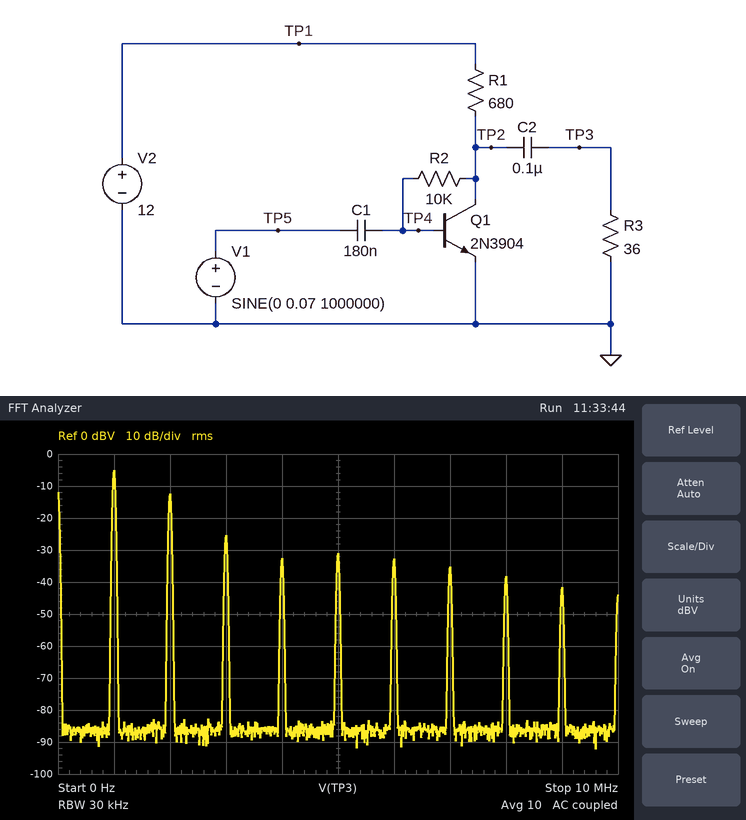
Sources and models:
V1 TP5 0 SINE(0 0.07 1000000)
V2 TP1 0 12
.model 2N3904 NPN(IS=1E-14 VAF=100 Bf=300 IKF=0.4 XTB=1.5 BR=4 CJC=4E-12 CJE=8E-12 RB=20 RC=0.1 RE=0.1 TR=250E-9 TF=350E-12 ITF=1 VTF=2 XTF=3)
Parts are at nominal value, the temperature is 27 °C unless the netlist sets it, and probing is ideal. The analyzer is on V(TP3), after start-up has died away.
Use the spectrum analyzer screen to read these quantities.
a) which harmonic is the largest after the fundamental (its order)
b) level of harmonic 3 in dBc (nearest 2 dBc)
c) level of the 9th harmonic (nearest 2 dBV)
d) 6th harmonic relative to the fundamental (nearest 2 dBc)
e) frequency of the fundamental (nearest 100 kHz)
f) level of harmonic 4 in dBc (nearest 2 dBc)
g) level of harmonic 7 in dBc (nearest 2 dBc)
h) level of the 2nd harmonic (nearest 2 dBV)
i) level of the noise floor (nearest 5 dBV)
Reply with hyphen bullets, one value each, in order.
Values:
- 2
- -20 dBc
- -42 dBV
- -28 dBc
- 1.0 MHz
- -28 dBc
- -30 dBc
- -12 dBV
- -85 dBV
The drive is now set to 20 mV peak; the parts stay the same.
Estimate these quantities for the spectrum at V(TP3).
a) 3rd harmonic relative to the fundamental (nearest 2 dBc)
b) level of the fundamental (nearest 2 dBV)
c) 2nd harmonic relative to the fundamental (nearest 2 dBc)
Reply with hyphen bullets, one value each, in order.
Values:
- -40 dBc
- -12 dBV
- -16 dBc
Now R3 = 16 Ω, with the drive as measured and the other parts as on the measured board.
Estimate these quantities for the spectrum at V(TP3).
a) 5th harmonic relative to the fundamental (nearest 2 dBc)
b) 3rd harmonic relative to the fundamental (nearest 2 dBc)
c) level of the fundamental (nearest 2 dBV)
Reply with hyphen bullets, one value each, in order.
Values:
- -44 dBc
- -18 dBc
- -12 dBV
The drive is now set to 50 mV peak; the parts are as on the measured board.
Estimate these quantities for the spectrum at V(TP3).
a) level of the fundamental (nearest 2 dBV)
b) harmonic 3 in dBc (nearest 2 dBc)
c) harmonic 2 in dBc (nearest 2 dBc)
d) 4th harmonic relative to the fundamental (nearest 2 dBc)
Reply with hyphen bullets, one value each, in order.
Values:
- -6 dBV
- -24 dBc
- -10 dBc
- -42 dBc
